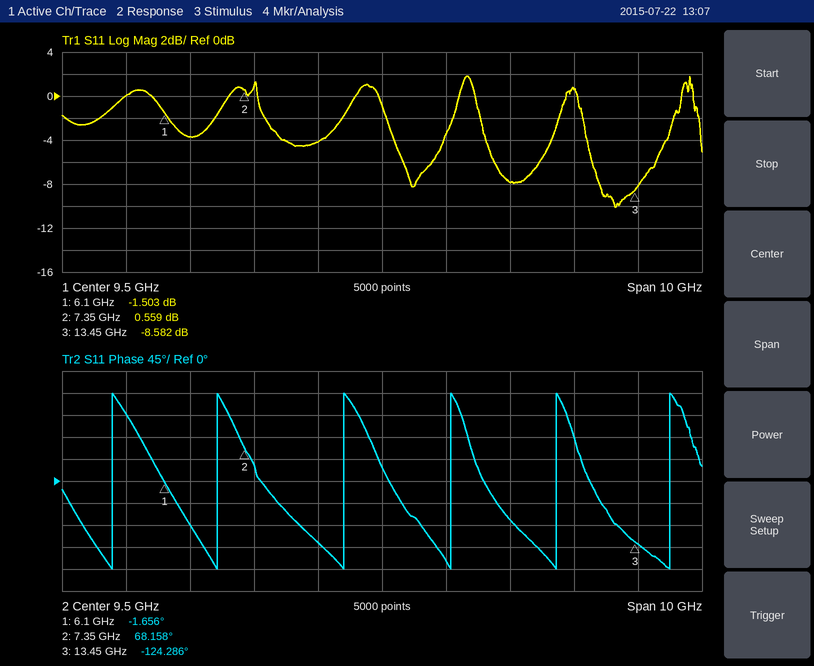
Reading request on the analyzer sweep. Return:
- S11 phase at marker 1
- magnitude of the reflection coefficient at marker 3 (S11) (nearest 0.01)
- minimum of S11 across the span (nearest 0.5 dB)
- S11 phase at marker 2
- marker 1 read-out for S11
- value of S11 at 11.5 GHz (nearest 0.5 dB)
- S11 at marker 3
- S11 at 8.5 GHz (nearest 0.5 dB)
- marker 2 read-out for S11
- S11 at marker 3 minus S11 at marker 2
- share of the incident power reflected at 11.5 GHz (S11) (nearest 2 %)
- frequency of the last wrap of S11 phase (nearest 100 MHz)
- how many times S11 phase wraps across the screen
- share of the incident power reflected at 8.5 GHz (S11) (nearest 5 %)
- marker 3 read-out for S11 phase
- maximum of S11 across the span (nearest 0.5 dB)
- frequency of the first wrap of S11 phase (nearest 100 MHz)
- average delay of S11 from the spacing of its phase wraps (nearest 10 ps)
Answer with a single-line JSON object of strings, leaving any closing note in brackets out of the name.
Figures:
{"S11 phase at marker 1": "-1.656°", "magnitude of the reflection coefficient at marker 3 (S11)": "0.37", "minimum of S11 across the span": "-10.0 dB", "S11 phase at marker 2": "68.158°", "marker 1 read-out for S11": "-1.503 dB", "value of S11 at 11.5 GHz": "-8.0 dB", "S11 at marker 3": "-8.582 dB", "S11 at 8.5 GHz": "-4.0 dB", "marker 2 read-out for S11": "0.559 dB", "S11 at marker 3 minus S11 at marker 2": "-9.141 dB", "share of the incident power reflected at 11.5 GHz (S11)": "16 %", "frequency of the last wrap of S11 phase": "14.0 GHz", "how many times S11 phase wraps across the screen": "6", "share of the incident power reflected at 8.5 GHz (S11)": "40 %", "marker 3 read-out for S11 phase": "-124.286°", "maximum of S11 across the span": "2.0 dB", "frequency of the first wrap of S11 phase": "5.3 GHz", "average delay of S11 from the spacing of its phase wraps": "570 ps"}
